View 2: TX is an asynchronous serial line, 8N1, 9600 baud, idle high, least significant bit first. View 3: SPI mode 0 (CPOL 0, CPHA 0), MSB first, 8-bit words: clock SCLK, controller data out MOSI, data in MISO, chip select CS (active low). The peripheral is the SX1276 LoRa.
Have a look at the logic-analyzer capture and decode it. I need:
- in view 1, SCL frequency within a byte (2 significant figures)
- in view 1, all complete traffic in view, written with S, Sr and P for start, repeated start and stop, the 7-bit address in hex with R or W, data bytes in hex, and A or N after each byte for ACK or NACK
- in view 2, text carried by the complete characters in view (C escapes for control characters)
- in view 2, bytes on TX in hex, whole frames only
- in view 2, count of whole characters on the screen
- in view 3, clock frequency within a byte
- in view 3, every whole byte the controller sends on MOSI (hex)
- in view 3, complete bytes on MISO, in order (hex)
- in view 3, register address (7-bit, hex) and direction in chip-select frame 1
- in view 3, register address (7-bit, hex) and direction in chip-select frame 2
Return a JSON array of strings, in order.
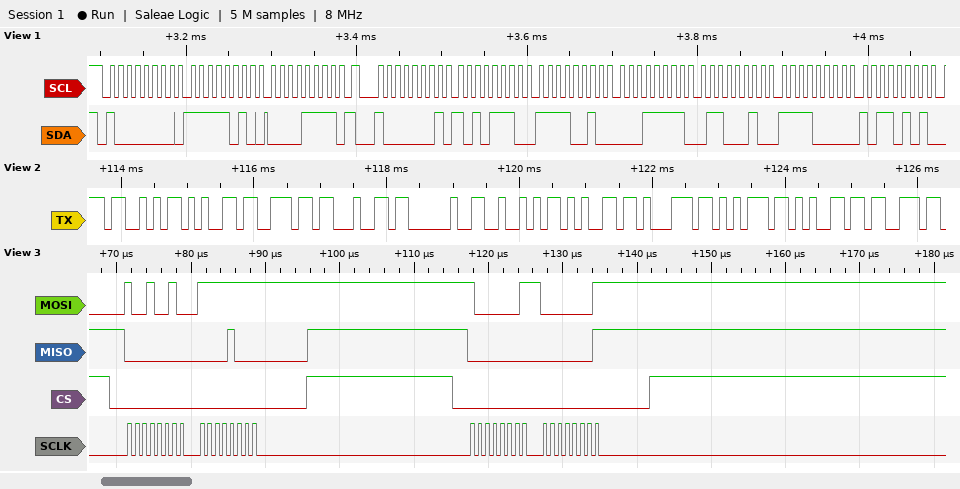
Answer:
["100 kHz", "S 40W A FA A 0F A Sr 40R A AE A F2 A 1F A 62 A F0 A B5 A", "\"Send Reques\"", "53 65 6E 64 20 52 65 71 75 65 73", "11", "1 MHz", "0x92 0xFF 0x81 0x01", "0x00 0x08 0x00 0x01", "0x12 write", "0x01 write"]
